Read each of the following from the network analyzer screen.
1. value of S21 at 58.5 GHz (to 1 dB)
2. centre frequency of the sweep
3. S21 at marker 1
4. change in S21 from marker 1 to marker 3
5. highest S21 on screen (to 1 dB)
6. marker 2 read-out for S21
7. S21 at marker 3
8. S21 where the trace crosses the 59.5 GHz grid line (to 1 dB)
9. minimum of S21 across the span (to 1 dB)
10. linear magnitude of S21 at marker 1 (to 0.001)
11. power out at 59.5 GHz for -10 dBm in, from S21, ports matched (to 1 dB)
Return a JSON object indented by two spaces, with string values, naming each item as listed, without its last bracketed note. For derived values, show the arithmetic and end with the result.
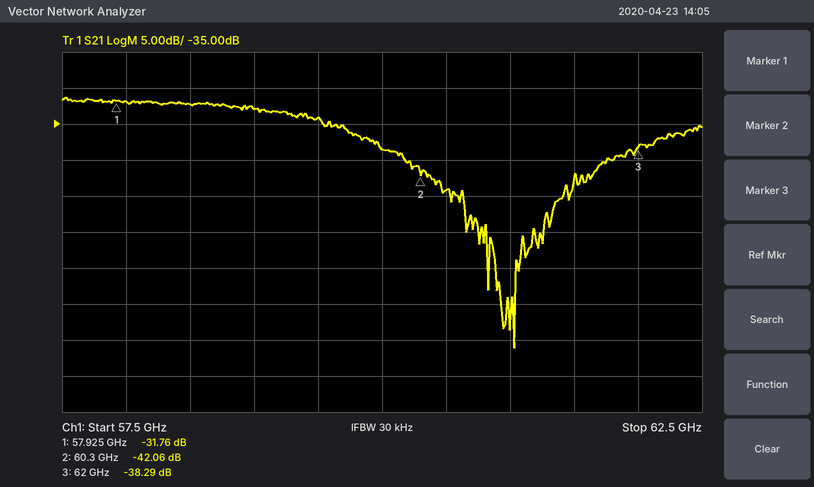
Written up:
{
  "value of S21 at 58.5 GHz": "-32 dB",
  "centre frequency of the sweep": "60 GHz",
  "S21 at marker 1": "-31.76 dB",
  "change in S21 from marker 1 to marker 3": "-38.29 − (-31.76) = -6.53 dB",
  "highest S21 on screen": "-31 dB",
  "marker 2 read-out for S21": "-42.06 dB",
  "S21 at marker 3": "-38.29 dB",
  "S21 where the trace crosses the 59.5 GHz grid line": "-34 dB",
  "minimum of S21 across the span": "-66 dB",
  "linear magnitude of S21 at marker 1": "10^(-31.76/20) ≈ 0.026",
  "power out at 59.5 GHz for -10 dBm in, from S21, ports matched": "-10 dBm + (-34 dB) = -44 dBm"
}
